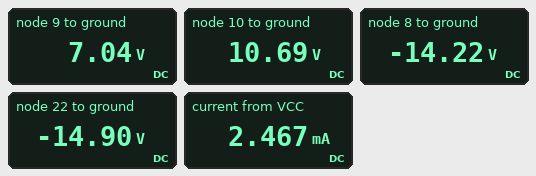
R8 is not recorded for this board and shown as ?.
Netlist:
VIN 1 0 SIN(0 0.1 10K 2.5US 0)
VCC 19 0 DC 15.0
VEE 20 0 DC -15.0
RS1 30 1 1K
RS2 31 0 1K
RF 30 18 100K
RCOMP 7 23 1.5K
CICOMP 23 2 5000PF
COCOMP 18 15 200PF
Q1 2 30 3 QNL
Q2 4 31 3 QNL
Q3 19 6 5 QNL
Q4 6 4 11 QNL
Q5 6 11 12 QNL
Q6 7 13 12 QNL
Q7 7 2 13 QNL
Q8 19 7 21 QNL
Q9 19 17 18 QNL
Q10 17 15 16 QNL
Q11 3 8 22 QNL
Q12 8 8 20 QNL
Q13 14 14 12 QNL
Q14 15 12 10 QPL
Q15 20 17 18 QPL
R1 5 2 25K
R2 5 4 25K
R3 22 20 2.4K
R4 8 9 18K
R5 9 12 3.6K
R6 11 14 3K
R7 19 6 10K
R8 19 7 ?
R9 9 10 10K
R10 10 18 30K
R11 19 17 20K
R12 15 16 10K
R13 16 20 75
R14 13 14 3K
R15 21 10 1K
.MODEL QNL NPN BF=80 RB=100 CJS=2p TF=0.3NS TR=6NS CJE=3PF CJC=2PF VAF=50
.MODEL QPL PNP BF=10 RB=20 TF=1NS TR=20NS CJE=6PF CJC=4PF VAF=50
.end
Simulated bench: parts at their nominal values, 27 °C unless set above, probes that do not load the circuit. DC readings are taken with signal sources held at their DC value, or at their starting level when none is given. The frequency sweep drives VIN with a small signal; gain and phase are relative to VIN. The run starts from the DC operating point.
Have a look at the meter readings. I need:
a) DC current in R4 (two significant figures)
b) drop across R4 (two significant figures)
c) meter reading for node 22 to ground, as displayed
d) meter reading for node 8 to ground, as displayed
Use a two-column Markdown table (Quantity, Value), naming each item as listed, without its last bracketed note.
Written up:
| Quantity | Value |
|---|---|
| DC current in R4 | 1.2 mA |
| drop across R4 | 21 V |
| meter reading for node 22 to ground, as displayed | -14.90 V |
| meter reading for node 8 to ground, as displayed | -14.22 V |
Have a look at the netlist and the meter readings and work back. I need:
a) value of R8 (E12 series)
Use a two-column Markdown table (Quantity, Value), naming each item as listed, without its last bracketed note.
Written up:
| Quantity | Value |
|---|---|
| value of R8 | 4.7 kΩ |
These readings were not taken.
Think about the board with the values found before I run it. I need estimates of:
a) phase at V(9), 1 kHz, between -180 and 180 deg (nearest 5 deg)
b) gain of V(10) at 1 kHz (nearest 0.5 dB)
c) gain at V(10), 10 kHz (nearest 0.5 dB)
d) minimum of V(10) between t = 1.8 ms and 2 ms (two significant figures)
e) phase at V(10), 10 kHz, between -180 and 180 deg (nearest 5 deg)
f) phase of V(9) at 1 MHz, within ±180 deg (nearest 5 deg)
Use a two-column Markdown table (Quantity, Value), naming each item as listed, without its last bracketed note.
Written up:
| Quantity | Value |
|---|---|
| phase at V(9), 1 kHz, between -180 and 180 deg | 170 deg |
| gain of V(10) at 1 kHz | 6.5 dB |
| gain at V(10), 10 kHz | 2.5 dB |
| minimum of V(10) between t = 1.8 ms and 2 ms | 11 V |
| phase at V(10), 10 kHz, between -180 and 180 deg | 105 deg |
| phase of V(9) at 1 MHz, within ±180 deg | 30 deg |
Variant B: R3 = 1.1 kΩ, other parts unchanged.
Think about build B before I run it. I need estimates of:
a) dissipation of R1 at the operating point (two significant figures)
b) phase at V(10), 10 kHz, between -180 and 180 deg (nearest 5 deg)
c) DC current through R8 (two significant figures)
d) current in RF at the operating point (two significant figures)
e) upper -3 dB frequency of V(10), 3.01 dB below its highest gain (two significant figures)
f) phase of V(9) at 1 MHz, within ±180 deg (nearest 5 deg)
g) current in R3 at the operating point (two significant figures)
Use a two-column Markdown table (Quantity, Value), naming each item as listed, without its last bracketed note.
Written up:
| Quantity | Value |
|---|---|
| dissipation of R1 at the operating point | 30 µW |
| phase at V(10), 10 kHz, between -180 and 180 deg | 125 deg |
| DC current through R8 | 610 µA |
| current in RF at the operating point | 1.5 µA |
| upper -3 dB frequency of V(10), 3.01 dB below its highest gain | 5.3 MHz |
| phase of V(9) at 1 MHz, within ±180 deg | 35 deg |
| current in R3 at the operating point | 72 µA |
